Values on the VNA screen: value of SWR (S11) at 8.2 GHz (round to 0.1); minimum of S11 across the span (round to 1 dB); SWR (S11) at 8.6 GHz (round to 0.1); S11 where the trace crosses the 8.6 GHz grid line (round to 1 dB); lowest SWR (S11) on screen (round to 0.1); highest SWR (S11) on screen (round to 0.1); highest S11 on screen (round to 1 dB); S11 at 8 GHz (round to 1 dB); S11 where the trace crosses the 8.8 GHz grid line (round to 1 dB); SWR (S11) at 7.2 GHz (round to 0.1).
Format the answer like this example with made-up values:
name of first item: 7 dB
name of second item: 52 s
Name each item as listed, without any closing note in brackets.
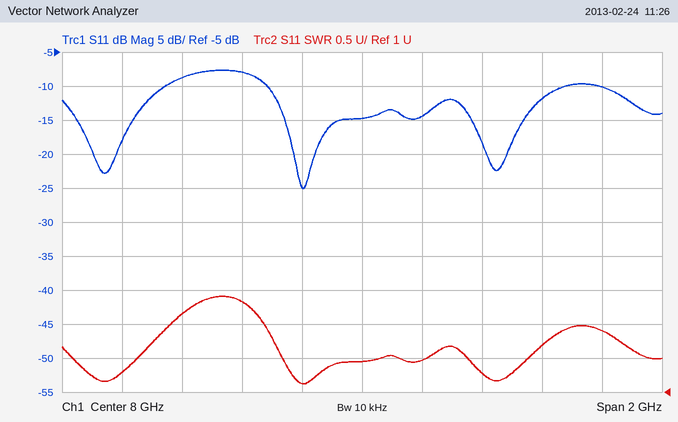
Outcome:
value of SWR (S11) at 8.2 GHz: 1.5
minimum of S11 across the span: -25 dB
SWR (S11) at 8.6 GHz: 1.7
S11 where the trace crosses the 8.6 GHz grid line: -12 dB
lowest SWR (S11) on screen: 1.1
highest SWR (S11) on screen: 2.4
highest S11 on screen: -8 dB
S11 at 8 GHz: -15 dB
S11 where the trace crosses the 8.8 GHz grid line: -10 dB
SWR (S11) at 7.2 GHz: 1.3
